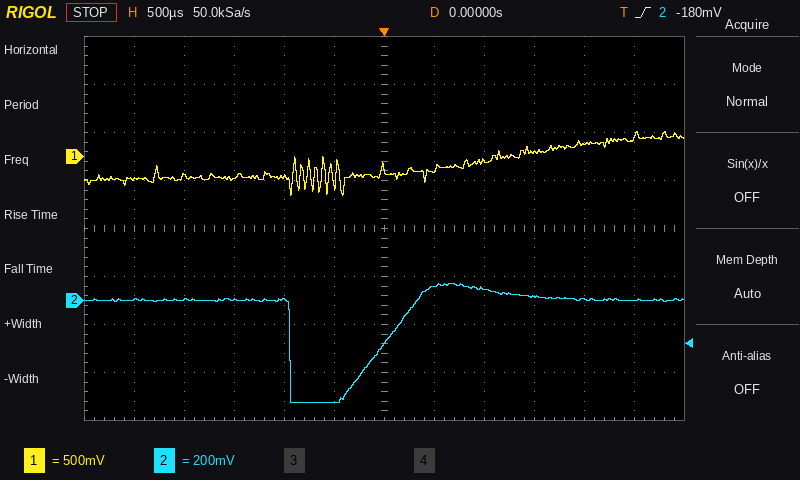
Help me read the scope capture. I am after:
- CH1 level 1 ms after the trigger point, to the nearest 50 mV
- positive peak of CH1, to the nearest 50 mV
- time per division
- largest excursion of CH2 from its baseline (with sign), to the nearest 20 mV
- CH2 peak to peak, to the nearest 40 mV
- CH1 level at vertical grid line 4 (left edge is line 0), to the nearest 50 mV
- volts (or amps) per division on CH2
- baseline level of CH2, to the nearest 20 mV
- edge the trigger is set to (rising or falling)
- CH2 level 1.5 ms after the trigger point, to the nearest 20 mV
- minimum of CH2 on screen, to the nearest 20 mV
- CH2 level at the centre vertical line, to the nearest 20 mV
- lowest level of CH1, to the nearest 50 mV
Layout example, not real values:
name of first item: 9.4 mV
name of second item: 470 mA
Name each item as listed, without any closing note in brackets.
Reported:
CH1 level 1 ms after the trigger point, to the nearest 50 mV: -50 mV
positive peak of CH1, to the nearest 50 mV: 250 mV
time per division: 500 µs
largest excursion of CH2 from its baseline (with sign), to the nearest 20 mV: -420 mV
CH2 peak to peak, to the nearest 40 mV: 480 mV
CH1 level at vertical grid line 4 (left edge is line 0), to the nearest 50 mV: -200 mV
volts (or amps) per division on CH2: 200 mV
baseline level of CH2, to the nearest 20 mV: 0 mV
edge the trigger is set to: rising
CH2 level 1.5 ms after the trigger point, to the nearest 20 mV: 20 mV
minimum of CH2 on screen, to the nearest 20 mV: -420 mV
CH2 level at the centre vertical line, to the nearest 20 mV: -180 mV
lowest level of CH1, to the nearest 50 mV: -400 mV
